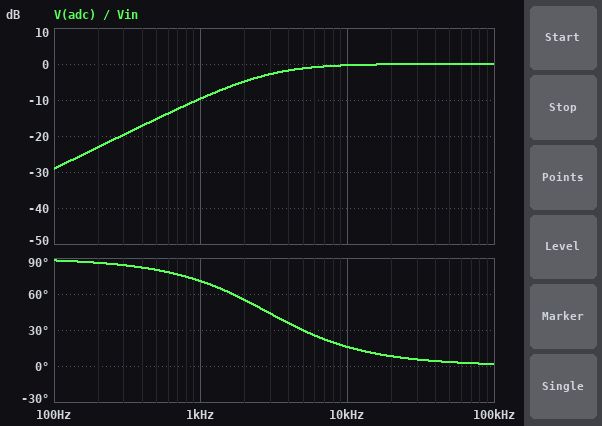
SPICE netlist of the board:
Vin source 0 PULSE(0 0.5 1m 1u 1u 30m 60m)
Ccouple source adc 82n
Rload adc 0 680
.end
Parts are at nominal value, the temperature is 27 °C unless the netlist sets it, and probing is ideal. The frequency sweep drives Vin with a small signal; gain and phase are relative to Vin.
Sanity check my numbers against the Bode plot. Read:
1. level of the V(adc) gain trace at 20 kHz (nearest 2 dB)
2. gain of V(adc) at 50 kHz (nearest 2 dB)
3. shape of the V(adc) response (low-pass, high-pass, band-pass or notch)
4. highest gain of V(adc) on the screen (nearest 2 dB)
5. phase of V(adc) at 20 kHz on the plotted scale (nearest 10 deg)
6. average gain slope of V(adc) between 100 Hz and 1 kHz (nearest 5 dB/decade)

0 dB
0 dB
high-pass
0 dB
10 deg
20 dB/decade
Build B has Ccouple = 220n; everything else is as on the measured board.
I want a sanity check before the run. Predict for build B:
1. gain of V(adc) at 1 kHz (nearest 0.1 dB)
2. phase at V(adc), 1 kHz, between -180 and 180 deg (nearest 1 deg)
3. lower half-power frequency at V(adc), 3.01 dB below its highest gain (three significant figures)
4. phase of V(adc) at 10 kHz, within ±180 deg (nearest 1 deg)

-3.3 dB
47 deg
1.06 kHz
6 deg
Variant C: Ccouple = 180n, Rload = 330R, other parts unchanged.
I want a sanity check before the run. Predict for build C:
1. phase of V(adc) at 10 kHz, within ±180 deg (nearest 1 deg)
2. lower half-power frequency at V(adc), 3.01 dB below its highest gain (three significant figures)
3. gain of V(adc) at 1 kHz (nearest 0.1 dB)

15 deg
2.68 kHz
-9.1 dB
